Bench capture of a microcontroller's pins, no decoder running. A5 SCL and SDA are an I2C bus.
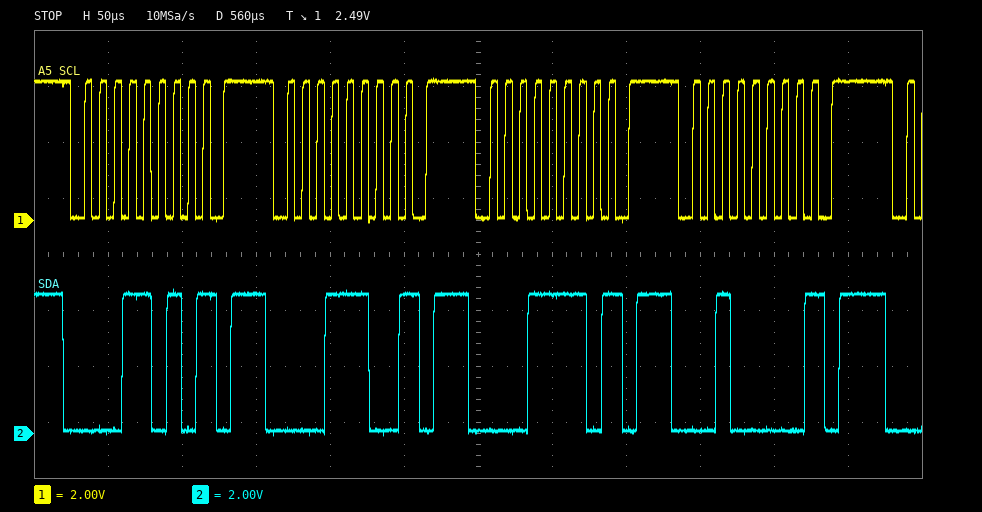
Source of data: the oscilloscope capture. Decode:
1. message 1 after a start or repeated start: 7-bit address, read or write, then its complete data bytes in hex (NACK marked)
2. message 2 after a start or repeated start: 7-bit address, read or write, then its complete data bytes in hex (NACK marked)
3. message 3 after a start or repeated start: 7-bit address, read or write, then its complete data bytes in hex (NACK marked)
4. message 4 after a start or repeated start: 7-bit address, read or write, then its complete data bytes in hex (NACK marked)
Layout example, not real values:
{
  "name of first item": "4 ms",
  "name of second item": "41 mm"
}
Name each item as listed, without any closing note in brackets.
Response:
{
  "message 1 after a start or repeated start: 7-bit address, read or write, then its complete data bytes in hex": "0x0D write NACK",
  "message 2 after a start or repeated start: 7-bit address, read or write, then its complete data bytes in hex": "0x0E write NACK",
  "message 3 after a start or repeated start: 7-bit address, read or write, then its complete data bytes in hex": "0x0F write NACK",
  "message 4 after a start or repeated start: 7-bit address, read or write, then its complete data bytes in hex": "0x10 write NACK"
}
